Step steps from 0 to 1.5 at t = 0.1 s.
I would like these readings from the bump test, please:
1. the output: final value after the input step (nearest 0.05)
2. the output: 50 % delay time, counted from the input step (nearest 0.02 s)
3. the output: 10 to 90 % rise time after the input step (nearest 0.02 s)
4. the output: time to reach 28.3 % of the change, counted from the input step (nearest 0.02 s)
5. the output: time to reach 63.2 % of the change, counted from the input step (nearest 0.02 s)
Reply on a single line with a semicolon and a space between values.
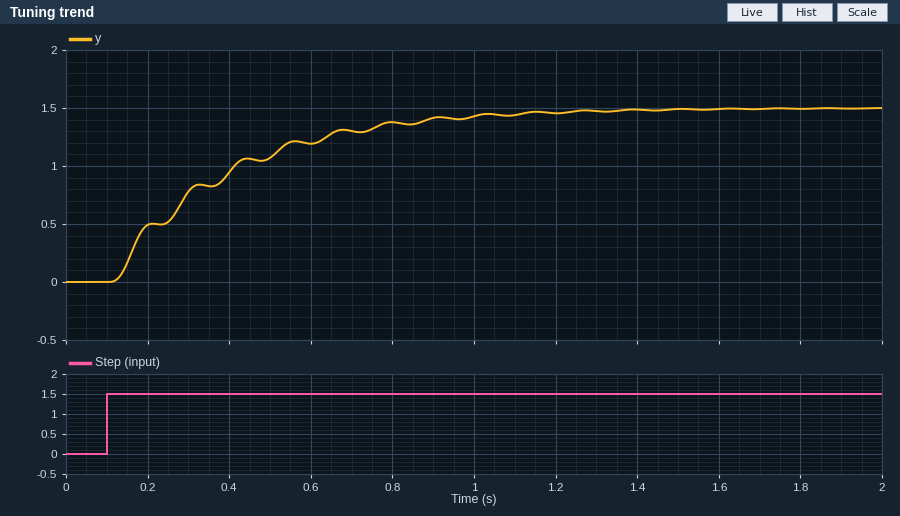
1.50; 0.20 s; 0.62 s; 0.08 s; 0.30 s
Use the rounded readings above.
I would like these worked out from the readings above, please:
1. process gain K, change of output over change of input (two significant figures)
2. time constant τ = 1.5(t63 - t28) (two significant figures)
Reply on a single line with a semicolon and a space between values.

1.0; 0.33 s
